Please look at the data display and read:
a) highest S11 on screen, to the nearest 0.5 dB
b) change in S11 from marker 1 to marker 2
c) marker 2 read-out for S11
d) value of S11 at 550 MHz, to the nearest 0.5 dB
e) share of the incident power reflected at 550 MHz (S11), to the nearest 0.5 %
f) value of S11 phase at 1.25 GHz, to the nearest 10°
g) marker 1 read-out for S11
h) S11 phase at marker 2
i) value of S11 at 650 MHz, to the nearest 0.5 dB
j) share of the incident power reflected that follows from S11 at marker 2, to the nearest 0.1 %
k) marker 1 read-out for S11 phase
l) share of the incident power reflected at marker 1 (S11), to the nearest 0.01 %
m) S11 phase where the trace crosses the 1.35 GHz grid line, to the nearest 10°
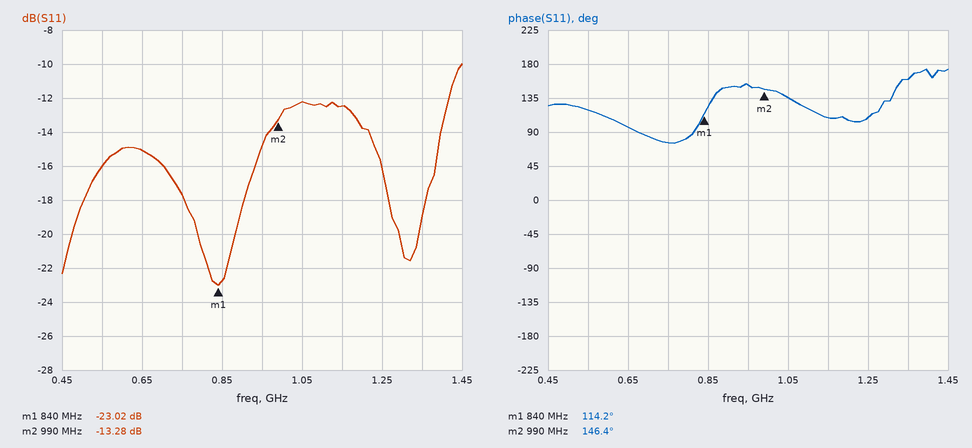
-10.0 dB
9.74 dB
-13.28 dB
-16.0 dB
2.5 %
110°
-23.02 dB
146.4°
-15.0 dB
4.7 %
114.2°
0.50 %
160°
